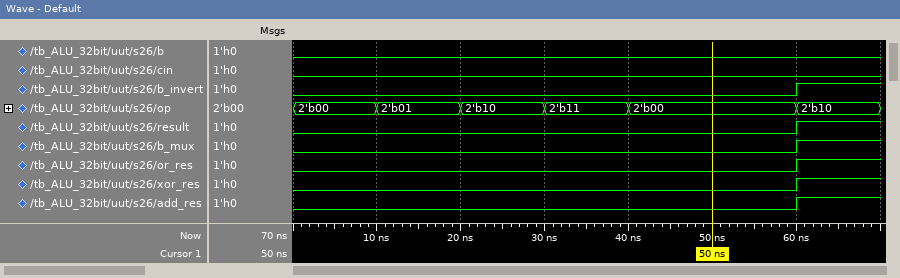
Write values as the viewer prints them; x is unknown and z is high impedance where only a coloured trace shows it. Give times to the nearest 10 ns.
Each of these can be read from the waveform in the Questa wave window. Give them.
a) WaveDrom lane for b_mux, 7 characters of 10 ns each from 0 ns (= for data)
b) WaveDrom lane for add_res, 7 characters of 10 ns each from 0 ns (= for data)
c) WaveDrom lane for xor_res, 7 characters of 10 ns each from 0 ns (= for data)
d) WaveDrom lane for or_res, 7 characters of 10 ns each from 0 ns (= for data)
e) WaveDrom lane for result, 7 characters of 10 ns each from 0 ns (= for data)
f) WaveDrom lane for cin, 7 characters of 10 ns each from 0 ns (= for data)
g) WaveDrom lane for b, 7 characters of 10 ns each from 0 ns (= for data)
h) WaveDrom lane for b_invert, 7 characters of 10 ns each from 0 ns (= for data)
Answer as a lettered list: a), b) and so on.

a) {name: 'b_mux', wave: '0.....1'}
b) {name: 'add_res', wave: '0.....1'}
c) {name: 'xor_res', wave: '0.....1'}
d) {name: 'or_res', wave: '0.....1'}
e) {name: 'result', wave: '0.....1'}
f) {name: 'cin', wave: '0......'}
g) {name: 'b', wave: '0......'}
h) {name: 'b_invert', wave: '0.....1'}
